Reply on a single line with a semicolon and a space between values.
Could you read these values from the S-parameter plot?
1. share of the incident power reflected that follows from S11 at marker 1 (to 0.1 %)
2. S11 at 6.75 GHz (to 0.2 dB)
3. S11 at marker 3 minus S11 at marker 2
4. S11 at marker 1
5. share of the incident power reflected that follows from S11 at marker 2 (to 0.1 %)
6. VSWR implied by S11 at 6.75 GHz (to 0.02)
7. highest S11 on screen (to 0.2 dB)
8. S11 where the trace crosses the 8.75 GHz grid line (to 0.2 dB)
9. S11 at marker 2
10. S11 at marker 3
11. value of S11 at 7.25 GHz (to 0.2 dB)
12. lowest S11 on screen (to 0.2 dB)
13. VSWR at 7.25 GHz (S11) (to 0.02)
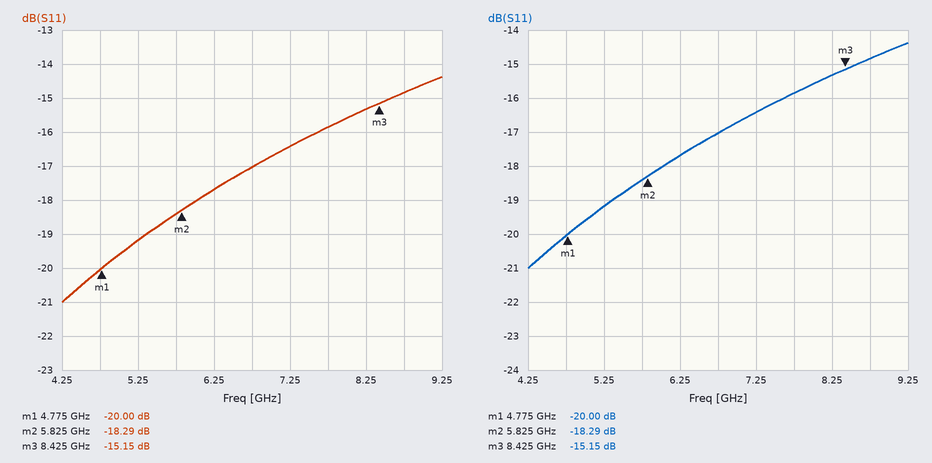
1.0 %; -17.0 dB; 3.14 dB; -20.00 dB; 1.5 %; 1.32; -14.4 dB; -14.8 dB; -18.29 dB; -15.15 dB; -16.4 dB; -21.0 dB; 1.36
